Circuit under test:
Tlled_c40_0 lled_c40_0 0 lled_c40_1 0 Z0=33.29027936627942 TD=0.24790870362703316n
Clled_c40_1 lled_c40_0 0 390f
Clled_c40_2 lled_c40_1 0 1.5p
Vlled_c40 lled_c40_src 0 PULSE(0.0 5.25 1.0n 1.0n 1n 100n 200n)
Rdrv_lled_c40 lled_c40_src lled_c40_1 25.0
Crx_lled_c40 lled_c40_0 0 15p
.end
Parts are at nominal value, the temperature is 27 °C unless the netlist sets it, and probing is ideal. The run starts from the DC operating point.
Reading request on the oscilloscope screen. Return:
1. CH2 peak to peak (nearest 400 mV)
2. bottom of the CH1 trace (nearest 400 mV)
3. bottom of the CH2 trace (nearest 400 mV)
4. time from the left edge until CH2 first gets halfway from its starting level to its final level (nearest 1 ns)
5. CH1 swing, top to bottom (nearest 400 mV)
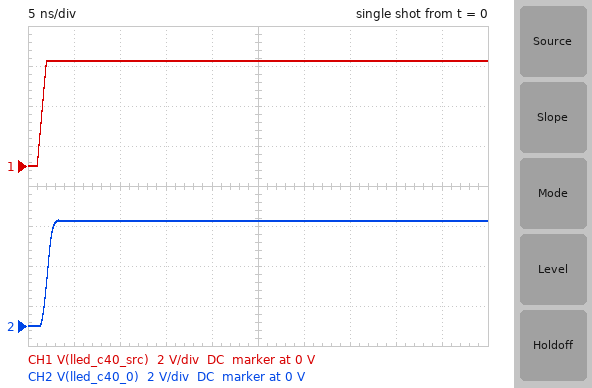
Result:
5.2 V
0 V
0 V
2 ns
5.2 V
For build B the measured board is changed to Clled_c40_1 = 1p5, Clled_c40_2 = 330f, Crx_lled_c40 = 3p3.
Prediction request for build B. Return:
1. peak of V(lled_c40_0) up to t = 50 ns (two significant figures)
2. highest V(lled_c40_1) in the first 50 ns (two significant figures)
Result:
5.5 V
5.4 V
